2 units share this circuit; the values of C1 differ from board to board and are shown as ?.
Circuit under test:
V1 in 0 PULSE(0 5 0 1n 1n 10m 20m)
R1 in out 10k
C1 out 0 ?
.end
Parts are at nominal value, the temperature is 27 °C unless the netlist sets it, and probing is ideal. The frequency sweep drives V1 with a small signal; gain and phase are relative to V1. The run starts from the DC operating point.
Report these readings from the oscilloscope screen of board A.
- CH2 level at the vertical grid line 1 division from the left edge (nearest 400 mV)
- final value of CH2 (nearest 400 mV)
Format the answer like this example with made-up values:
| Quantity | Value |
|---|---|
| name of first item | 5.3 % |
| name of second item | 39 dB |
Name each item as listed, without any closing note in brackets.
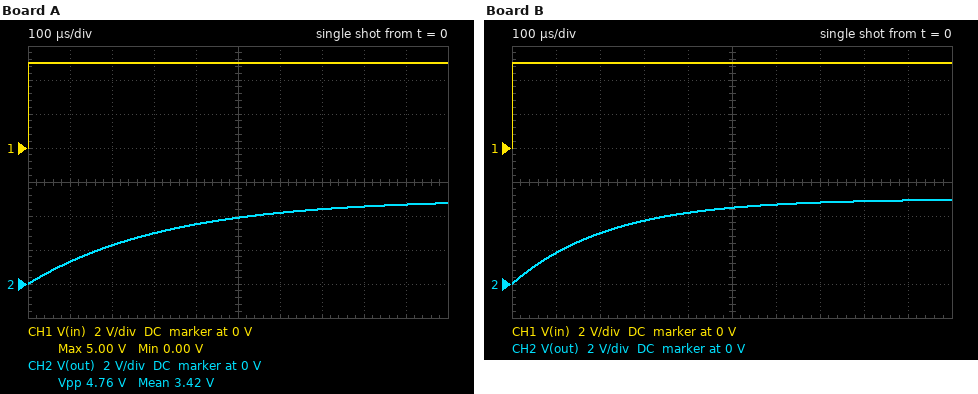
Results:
| Quantity | Value |
|---|---|
| CH2 level at the vertical grid line 1 division from the left edge | 1.2 V |
| final value of CH2 | 4.8 V |
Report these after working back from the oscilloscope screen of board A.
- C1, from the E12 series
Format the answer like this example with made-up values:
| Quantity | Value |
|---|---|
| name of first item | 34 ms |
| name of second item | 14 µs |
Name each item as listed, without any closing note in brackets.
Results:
| Quantity | Value |
|---|---|
| C1, from the E12 series | 33 nF |
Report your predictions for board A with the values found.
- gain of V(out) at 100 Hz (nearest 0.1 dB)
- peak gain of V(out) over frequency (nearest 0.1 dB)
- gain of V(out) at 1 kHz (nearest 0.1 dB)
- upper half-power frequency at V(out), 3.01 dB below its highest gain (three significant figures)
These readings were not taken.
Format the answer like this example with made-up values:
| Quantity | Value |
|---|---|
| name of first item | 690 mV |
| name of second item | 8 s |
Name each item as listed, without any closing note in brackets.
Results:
| Quantity | Value |
|---|---|
| gain of V(out) at 100 Hz | -0.2 dB |
| peak gain of V(out) over frequency | 0 dB |
| gain of V(out) at 1 kHz | -7.2 dB |
| upper half-power frequency at V(out), 3.01 dB below its highest gain | 482 Hz |
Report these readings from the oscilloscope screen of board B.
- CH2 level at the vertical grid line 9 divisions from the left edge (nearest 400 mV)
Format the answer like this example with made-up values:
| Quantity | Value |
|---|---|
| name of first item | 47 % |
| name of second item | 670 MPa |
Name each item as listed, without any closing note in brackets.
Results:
| Quantity | Value |
|---|---|
| CH2 level at the vertical grid line 9 divisions from the left edge | 4.8 V |
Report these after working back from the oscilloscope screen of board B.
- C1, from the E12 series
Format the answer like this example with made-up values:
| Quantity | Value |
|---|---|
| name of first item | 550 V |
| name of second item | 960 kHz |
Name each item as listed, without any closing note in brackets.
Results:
| Quantity | Value |
|---|---|
| C1, from the E12 series | 22 nF |
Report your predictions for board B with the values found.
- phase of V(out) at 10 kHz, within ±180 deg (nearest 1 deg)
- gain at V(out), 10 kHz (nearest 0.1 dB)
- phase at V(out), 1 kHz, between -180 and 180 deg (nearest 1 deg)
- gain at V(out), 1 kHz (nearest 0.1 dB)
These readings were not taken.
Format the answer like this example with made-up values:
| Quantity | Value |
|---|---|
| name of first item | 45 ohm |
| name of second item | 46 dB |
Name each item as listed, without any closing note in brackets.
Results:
| Quantity | Value |
|---|---|
| phase of V(out) at 10 kHz, within ±180 deg | -86 deg |
| gain at V(out), 10 kHz | -22.8 dB |
| phase at V(out), 1 kHz, between -180 and 180 deg | -54 deg |
| gain at V(out), 1 kHz | -4.6 dB |
